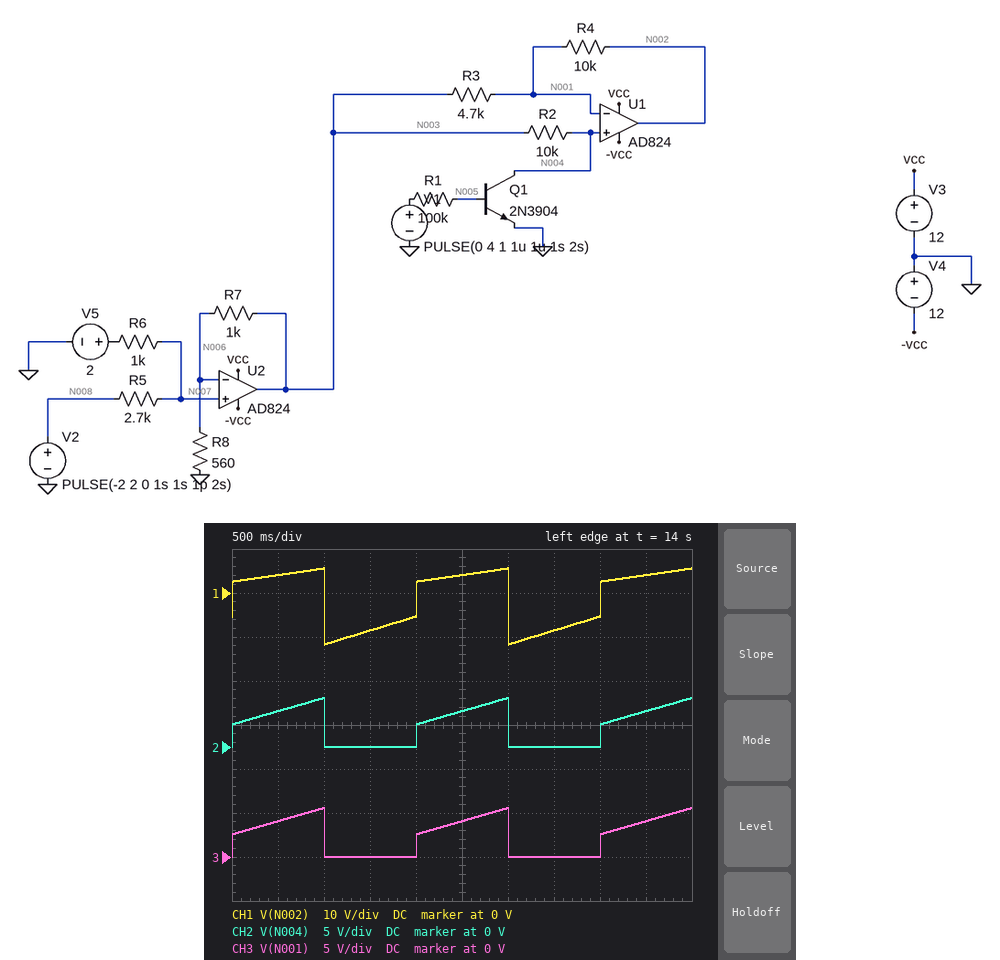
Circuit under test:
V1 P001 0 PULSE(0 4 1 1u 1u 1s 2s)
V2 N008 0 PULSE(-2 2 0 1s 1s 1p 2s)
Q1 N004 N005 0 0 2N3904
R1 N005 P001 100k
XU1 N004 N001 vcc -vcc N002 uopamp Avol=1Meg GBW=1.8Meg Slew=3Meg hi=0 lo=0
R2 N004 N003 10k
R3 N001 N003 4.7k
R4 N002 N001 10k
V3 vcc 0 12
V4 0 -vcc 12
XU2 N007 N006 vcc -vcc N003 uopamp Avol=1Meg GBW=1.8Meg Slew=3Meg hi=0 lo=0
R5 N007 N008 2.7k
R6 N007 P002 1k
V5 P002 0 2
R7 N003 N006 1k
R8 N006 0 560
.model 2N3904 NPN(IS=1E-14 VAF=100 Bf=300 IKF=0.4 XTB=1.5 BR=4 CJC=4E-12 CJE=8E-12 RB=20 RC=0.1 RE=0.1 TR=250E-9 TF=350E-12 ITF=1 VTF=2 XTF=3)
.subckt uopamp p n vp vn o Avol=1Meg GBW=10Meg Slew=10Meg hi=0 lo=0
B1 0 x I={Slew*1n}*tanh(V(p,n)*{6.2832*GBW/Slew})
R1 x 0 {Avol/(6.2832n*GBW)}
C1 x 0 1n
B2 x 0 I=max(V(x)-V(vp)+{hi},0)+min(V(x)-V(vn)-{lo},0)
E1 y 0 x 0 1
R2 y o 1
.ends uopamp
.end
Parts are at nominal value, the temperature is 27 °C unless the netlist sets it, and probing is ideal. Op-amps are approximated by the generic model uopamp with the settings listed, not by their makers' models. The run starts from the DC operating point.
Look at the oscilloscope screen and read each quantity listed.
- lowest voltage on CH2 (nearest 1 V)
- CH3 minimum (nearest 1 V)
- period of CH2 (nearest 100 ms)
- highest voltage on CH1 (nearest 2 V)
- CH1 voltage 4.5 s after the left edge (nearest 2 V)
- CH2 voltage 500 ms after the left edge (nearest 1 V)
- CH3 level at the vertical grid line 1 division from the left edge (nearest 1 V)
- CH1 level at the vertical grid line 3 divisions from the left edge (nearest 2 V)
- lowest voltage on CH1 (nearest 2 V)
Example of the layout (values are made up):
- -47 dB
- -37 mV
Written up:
- 0 V
- 0 V
- 2.0 s
- 6 V
- 4 V
- 4 V
- 4 V
- -8 V
- -12 V
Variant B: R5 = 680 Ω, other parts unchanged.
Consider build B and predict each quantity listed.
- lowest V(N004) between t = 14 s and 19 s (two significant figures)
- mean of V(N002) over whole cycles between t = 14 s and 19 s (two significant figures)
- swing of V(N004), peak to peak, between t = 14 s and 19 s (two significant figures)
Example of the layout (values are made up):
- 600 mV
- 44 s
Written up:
- -890 mV
- -1.2 V
- 6.5 V
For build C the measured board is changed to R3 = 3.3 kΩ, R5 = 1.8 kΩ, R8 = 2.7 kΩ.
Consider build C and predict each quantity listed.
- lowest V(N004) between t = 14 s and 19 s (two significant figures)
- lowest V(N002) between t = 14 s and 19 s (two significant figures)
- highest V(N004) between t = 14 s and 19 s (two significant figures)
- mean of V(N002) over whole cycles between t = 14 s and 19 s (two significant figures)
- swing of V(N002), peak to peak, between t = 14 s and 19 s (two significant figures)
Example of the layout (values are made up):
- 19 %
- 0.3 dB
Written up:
- 15 mV
- -8.2 V
- 2.8 V
- -1.7 V
- 11 V
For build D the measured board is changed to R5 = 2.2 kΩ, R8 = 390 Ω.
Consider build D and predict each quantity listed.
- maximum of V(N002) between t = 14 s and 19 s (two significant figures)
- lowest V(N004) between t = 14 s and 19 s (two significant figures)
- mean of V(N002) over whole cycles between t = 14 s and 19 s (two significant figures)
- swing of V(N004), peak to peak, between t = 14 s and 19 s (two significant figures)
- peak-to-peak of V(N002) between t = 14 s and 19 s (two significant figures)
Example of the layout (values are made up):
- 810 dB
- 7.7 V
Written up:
- 7.2 V
- 31 mV
- -2.5 V
- 7.1 V
- 19 V
